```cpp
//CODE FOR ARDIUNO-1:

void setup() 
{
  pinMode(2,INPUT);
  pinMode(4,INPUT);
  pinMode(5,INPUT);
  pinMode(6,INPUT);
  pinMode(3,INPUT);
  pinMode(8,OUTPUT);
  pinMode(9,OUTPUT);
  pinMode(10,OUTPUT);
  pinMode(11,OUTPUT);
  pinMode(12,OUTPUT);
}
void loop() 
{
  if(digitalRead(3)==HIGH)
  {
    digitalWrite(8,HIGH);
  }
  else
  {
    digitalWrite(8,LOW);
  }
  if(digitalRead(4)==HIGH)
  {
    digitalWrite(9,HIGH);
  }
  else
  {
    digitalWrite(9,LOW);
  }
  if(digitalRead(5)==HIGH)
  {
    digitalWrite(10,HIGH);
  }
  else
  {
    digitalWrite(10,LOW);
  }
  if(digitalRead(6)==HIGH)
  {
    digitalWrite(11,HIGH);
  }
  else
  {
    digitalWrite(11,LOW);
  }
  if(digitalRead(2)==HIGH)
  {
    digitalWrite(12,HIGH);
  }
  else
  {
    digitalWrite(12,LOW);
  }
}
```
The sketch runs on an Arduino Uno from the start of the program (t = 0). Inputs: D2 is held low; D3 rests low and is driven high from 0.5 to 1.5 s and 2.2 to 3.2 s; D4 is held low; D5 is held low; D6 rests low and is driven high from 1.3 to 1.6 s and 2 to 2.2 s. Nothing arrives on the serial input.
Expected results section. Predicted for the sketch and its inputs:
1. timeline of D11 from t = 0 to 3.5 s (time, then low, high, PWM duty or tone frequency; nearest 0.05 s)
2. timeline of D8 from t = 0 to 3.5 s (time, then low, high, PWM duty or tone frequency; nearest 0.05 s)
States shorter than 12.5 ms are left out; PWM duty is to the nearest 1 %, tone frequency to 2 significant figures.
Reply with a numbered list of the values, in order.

1. 0 s low; 1.3 s high; 1.6 s low; 2 s high; 2.2 s low
2. 0 s low; 0.5 s high; 1.5 s low; 2.2 s high; 3.2 s low
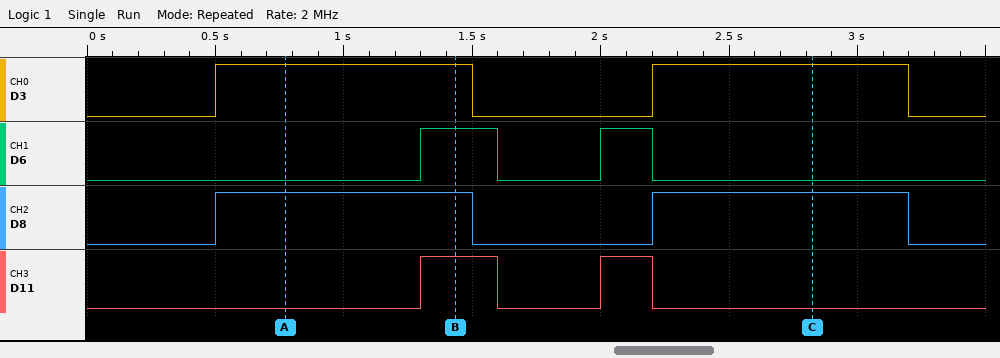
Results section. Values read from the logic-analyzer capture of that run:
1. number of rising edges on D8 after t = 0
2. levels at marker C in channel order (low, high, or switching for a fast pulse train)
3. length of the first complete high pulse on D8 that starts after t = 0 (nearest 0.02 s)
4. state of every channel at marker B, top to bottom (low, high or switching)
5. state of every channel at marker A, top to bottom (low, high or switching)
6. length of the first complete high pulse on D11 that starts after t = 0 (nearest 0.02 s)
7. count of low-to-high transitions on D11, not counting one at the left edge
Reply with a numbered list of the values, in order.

1. 2
2. D3 high, D6 low, D8 high, D11 low
3. 1.00 s
4. D3 high, D6 high, D8 high, D11 high
5. D3 high, D6 low, D8 high, D11 low
6. 0.30 s
7. 2
